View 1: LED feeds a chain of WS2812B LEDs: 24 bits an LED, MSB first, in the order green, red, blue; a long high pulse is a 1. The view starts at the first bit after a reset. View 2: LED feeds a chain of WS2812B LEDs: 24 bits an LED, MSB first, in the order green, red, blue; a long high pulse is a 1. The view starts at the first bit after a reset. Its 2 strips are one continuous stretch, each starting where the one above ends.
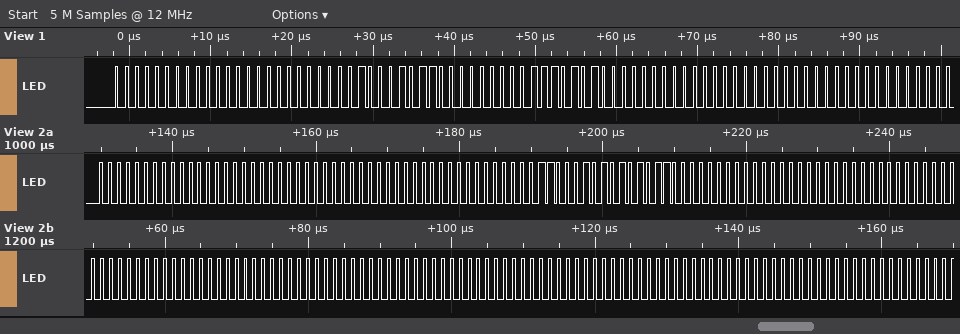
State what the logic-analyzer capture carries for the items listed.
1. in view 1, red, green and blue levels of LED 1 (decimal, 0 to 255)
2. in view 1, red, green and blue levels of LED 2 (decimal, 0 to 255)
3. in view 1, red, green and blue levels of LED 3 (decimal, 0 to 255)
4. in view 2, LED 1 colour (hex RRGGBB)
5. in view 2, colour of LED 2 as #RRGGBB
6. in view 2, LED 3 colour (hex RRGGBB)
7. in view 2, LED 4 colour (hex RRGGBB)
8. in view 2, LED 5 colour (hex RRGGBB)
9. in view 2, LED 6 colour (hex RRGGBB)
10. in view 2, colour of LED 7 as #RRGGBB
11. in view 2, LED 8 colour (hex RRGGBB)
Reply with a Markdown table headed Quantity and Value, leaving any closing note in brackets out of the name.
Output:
| Quantity | Value |
|---|---|
| in view 1, red, green and blue levels of LED 1 | 0, 0, 0 |
| in view 1, red, green and blue levels of LED 2 | 0, 139, 117 |
| in view 1, red, green and blue levels of LED 3 | 0, 0, 0 |
| in view 2, LED 1 colour | #000000 |
| in view 2, colour of LED 2 as #RRGGBB | #000000 |
| in view 2, LED 3 colour | #AB6200 |
| in view 2, LED 4 colour | #000000 |
| in view 2, LED 5 colour | #000000 |
| in view 2, LED 6 colour | #000000 |
| in view 2, colour of LED 7 as #RRGGBB | #000000 |
| in view 2, LED 8 colour | #000000 |
